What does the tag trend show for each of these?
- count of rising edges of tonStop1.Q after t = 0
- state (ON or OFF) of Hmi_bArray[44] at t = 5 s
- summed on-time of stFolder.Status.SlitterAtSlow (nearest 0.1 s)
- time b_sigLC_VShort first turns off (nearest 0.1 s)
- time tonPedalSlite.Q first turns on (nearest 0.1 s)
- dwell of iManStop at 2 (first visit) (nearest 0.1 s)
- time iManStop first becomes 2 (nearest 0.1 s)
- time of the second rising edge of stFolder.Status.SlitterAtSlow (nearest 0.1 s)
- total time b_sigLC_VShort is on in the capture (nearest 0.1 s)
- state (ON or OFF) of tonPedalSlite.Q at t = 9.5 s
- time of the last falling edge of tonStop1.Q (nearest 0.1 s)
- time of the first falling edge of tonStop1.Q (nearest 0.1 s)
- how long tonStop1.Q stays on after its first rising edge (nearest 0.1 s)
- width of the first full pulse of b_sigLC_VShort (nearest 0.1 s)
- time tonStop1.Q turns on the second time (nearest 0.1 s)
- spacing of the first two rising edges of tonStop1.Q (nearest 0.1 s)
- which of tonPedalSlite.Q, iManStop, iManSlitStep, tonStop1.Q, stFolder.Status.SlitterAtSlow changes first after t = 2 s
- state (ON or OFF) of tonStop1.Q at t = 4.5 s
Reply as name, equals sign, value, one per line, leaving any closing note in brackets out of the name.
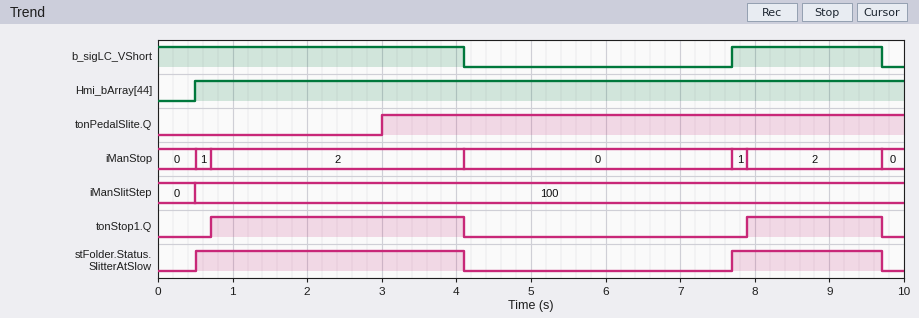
count of rising edges of tonStop1.Q after t = 0 = 2
state (ON or OFF) of Hmi_bArray[44] at t = 5 s = ON
summed on-time of stFolder.Status.SlitterAtSlow = 5.6 s
time b_sigLC_VShort first turns off = 4.1 s
time tonPedalSlite.Q first turns on = 3.0 s
dwell of iManStop at 2 (first visit) = 3.4 s
time iManStop first becomes 2 = 0.7 s
time of the second rising edge of stFolder.Status.SlitterAtSlow = 7.7 s
total time b_sigLC_VShort is on in the capture = 6.1 s
state (ON or OFF) of tonPedalSlite.Q at t = 9.5 s = ON
time of the last falling edge of tonStop1.Q = 9.7 s
time of the first falling edge of tonStop1.Q = 4.1 s
how long tonStop1.Q stays on after its first rising edge = 3.4 s
width of the first full pulse of b_sigLC_VShort = 2.0 s
time tonStop1.Q turns on the second time = 7.9 s
spacing of the first two rising edges of tonStop1.Q = 7.2 s
which of tonPedalSlite.Q, iManStop, iManSlitStep, tonStop1.Q, stFolder.Status.SlitterAtSlow changes first after t = 2 s = tonPedalSlite.Q
state (ON or OFF) of tonStop1.Q at t = 4.5 s = OFF
